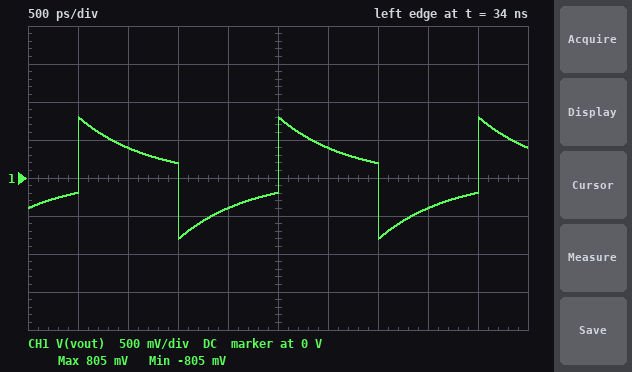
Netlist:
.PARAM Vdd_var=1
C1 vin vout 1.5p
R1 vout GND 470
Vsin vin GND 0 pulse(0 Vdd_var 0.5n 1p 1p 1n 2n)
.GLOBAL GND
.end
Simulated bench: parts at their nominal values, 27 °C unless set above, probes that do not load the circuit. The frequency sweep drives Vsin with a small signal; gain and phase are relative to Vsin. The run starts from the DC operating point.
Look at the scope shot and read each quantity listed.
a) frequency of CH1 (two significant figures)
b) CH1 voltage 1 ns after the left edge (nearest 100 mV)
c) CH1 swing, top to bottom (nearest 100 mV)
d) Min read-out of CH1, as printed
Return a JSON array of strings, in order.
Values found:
["500 MHz", "400 mV", "1.6 V", "-805 mV"]
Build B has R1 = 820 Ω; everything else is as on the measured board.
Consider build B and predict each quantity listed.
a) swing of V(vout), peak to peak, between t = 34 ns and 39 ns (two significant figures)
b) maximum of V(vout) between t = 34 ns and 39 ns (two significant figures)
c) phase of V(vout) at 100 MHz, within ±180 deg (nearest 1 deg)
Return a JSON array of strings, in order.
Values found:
["1.4 V", "690 mV", "52 deg"]
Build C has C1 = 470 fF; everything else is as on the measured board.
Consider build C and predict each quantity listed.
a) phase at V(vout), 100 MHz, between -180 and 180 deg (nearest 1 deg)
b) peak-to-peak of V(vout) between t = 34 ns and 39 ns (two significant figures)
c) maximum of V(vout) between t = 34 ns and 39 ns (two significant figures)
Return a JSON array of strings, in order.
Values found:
["82 deg", "2.0 V", "990 mV"]
